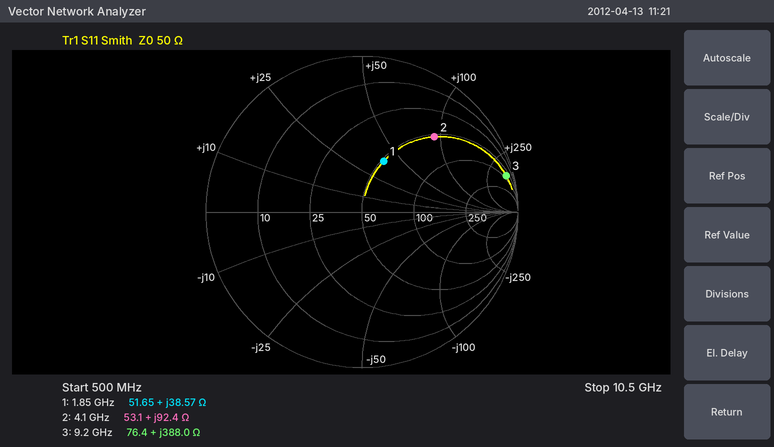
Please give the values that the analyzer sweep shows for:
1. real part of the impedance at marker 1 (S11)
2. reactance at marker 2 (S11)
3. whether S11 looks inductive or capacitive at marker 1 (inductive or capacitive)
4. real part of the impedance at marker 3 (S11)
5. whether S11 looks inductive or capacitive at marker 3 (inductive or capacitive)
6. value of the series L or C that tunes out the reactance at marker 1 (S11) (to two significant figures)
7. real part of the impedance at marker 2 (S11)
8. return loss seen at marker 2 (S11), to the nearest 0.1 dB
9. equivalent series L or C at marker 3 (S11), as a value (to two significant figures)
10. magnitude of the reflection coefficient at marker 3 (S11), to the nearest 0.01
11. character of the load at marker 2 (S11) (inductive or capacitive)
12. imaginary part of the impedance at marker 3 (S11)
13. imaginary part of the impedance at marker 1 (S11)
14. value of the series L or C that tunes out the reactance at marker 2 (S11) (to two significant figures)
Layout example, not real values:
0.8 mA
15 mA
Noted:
51.65 Ω
+92.4 Ω
inductive
76.4 Ω
inductive
2.2 pF
53.1 Ω
3.5 dB
6.7 nH
0.95
inductive
+388.0 Ω
+38.57 Ω
420 fF
